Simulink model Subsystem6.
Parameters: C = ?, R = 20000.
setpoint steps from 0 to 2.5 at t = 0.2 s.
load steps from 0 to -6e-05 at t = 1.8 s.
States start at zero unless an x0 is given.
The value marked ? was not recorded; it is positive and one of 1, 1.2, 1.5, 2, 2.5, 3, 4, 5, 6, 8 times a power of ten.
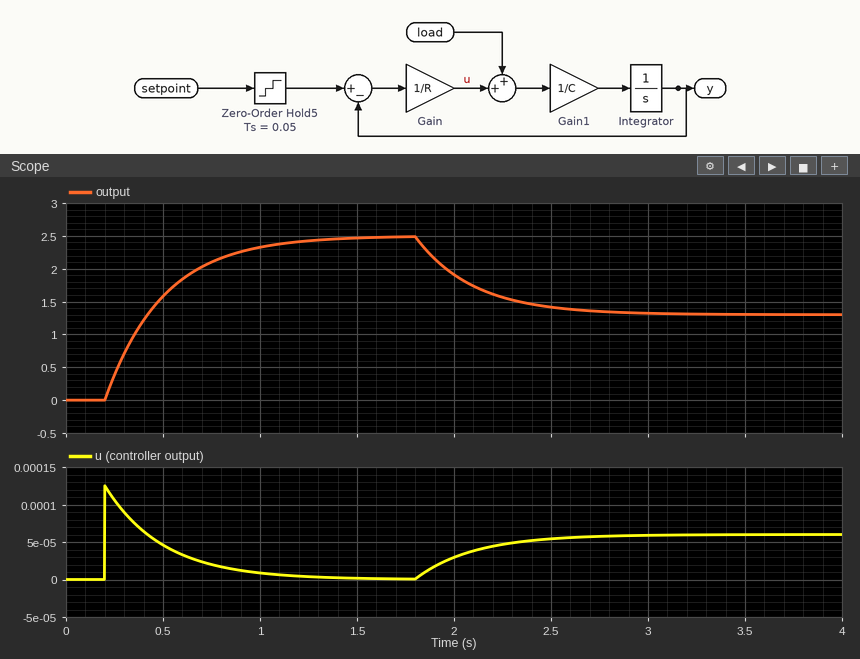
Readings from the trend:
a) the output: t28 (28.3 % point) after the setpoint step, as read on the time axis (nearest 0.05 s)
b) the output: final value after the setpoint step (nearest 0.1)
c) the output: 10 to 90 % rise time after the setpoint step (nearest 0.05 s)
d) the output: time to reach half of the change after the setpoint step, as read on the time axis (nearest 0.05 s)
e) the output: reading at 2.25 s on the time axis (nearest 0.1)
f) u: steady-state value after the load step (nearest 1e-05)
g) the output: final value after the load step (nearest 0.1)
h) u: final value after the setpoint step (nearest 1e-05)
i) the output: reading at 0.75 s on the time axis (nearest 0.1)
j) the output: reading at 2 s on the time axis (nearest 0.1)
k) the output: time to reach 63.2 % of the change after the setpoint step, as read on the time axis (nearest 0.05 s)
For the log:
0.30 s
2.5
0.65 s
0.40 s
1.6
0.00006
1.3
0.00000
2.1
1.9
0.50 s
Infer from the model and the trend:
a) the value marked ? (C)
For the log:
1.5e-05
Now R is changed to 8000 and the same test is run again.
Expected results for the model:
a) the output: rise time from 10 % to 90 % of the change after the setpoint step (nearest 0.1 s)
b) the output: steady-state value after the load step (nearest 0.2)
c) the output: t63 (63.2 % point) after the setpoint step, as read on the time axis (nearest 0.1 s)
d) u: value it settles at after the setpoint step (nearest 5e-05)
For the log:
0.3 s
2.0
0.3 s
0.00000
